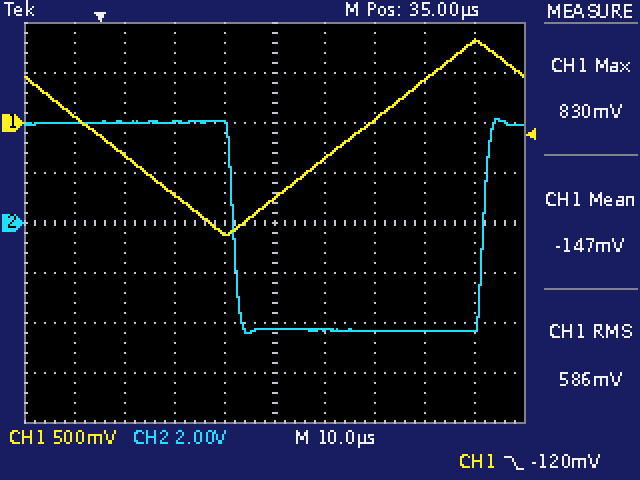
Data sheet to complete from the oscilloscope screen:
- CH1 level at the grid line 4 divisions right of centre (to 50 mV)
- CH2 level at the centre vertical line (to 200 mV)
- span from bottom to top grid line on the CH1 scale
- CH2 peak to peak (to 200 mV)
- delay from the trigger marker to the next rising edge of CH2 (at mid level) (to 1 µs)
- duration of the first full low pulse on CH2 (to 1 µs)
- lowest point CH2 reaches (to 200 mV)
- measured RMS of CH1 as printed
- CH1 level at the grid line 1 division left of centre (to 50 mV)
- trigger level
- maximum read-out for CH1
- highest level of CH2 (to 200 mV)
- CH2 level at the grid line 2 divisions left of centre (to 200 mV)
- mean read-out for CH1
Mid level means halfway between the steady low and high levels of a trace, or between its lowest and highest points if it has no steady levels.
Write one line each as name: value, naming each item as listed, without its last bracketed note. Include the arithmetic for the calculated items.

CH1 level at the grid line 4 divisions right of centre: 800 mV
CH2 level at the centre vertical line: -4.2 V
span from bottom to top grid line on the CH1 scale: 4 V
CH2 peak to peak: 4.2 V − (-4.4 V) = 8.6 V
delay from the trigger marker to the next rising edge of CH2 (at mid level): 77 µs
duration of the first full low pulse on CH2: 50 µs
lowest point CH2 reaches: -4.4 V
measured RMS of CH1 as printed: 586 mV
CH1 level at the grid line 1 division left of centre: -1.10 V
trigger level: -120 mV
maximum read-out for CH1: 830 mV
highest level of CH2: 4.2 V
CH2 level at the grid line 2 divisions left of centre: 4.0 V
mean read-out for CH1: -147 mV
